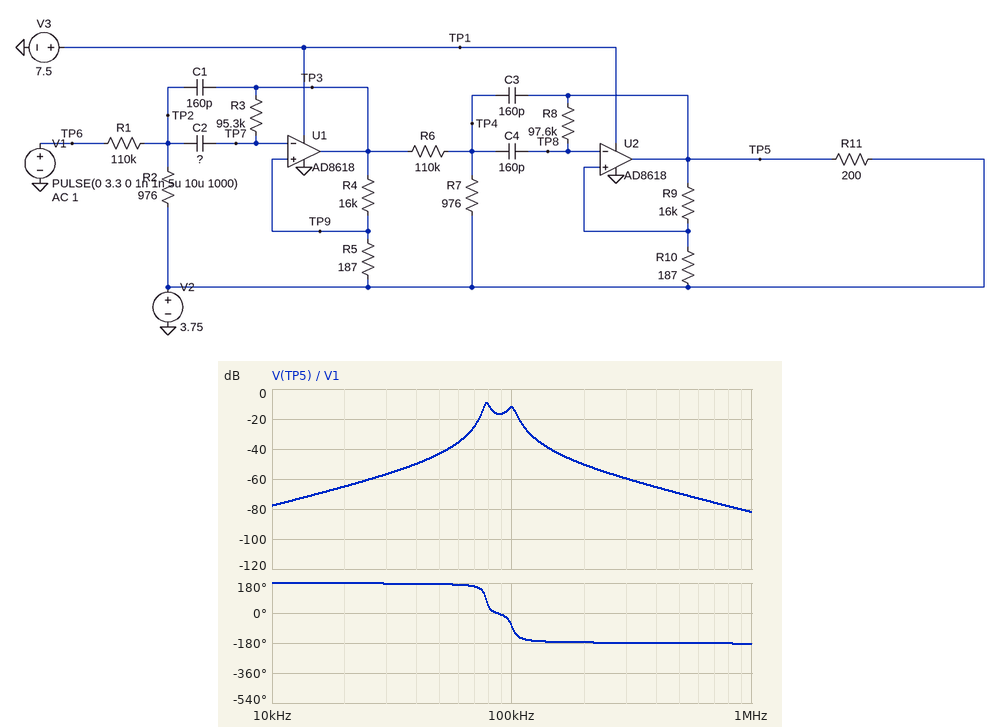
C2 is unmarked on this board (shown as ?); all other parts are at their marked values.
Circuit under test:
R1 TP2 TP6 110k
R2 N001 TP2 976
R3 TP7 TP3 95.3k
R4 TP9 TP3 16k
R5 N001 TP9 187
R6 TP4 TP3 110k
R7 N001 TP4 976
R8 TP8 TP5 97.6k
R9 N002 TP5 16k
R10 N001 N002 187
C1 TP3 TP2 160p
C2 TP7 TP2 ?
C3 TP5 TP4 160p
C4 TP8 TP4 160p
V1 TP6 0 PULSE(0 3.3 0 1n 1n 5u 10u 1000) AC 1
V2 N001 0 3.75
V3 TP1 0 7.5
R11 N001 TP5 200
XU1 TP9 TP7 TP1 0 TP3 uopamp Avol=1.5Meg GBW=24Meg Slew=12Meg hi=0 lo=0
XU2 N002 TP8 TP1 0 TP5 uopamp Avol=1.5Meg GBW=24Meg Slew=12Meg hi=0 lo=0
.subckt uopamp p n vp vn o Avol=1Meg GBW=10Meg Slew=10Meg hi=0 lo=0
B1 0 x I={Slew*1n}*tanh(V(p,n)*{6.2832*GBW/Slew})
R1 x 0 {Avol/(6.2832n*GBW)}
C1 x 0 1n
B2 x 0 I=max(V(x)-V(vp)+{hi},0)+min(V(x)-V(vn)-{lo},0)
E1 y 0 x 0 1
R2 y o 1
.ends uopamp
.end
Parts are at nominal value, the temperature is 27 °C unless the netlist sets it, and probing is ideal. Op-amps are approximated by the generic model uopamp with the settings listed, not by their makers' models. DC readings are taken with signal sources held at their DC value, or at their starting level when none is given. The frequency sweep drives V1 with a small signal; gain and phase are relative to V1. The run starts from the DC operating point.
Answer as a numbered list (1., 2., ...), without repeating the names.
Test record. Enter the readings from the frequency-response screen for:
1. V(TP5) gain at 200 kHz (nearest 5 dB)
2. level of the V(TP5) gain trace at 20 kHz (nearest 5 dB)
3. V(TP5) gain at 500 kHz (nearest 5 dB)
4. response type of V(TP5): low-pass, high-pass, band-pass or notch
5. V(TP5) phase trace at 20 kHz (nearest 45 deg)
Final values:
1. -50 dB
2. -65 dB
3. -70 dB
4. band-pass
5. 180 deg
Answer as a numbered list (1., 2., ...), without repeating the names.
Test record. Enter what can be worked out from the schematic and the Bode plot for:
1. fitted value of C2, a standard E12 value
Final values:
1. 270 pF
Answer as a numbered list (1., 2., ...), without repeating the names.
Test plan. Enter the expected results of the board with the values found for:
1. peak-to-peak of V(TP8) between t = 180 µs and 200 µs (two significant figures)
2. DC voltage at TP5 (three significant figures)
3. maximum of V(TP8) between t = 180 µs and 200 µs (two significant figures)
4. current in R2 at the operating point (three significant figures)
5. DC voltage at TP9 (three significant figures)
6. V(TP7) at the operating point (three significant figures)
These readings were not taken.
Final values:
1. 12 mV
2. 3.75 V
3. 3.8 V
4. 33.8 µA
5. 3.75 V
6. 3.75 V
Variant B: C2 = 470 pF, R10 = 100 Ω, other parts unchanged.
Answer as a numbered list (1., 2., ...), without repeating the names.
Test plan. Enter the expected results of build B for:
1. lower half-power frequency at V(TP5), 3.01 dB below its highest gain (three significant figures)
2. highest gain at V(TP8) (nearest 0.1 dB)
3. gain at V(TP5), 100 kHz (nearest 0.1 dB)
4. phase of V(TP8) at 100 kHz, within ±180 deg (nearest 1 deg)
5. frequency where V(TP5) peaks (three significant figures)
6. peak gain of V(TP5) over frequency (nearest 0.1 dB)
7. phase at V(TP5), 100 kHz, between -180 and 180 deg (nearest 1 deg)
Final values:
1. 58.3 kHz
2. -52.3 dB
3. -21.1 dB
4. -121 deg
5. 59.2 kHz
6. -8.8 dB
7. -87 deg
